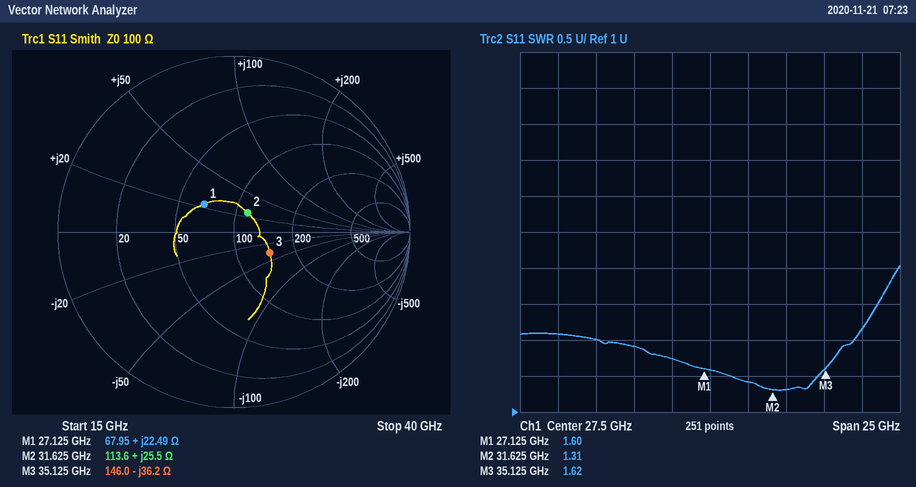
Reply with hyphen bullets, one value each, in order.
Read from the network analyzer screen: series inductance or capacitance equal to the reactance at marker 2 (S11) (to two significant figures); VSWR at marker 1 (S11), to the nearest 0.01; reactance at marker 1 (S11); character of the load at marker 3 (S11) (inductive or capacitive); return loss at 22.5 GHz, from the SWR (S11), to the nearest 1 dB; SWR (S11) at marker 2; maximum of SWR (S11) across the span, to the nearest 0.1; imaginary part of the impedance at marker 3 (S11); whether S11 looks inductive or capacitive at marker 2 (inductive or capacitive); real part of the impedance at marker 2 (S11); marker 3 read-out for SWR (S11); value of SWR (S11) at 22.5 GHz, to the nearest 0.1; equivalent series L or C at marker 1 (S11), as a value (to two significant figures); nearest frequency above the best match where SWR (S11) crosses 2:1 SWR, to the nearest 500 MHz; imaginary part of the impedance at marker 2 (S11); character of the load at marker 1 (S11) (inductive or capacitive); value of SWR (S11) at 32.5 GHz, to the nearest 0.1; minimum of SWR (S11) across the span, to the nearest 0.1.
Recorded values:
- 130 pH
- 1.60
- +22.49 Ω
- capacitive
- 10 dB
- 1.31
- 3.0
- -36.2 Ω
- inductive
- 113.6 Ω
- 1.62
- 1.9
- 130 pH
- 37.0 GHz
- +25.5 Ω
- inductive
- 1.3
- 1.3
